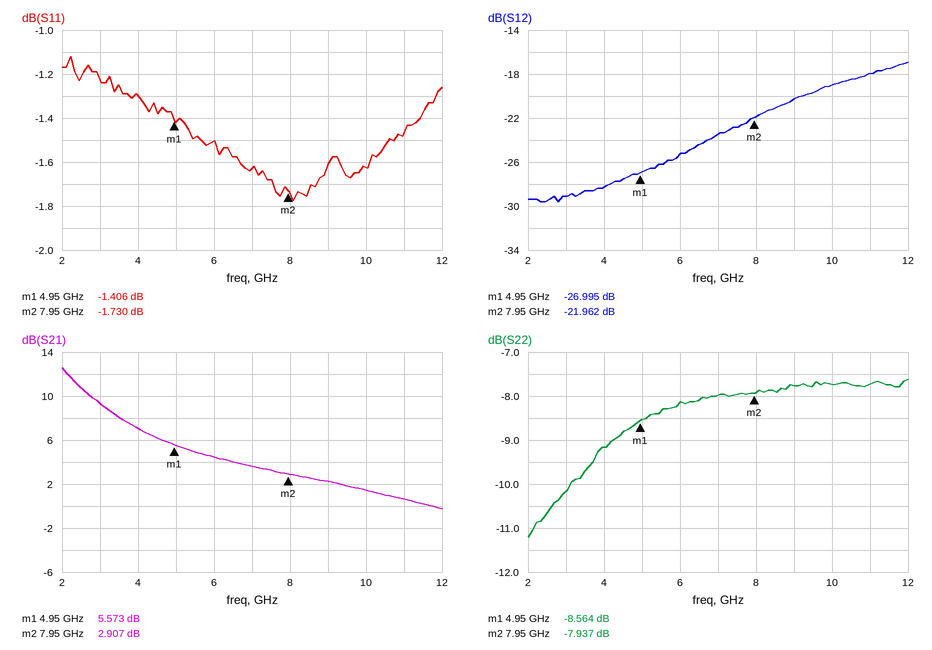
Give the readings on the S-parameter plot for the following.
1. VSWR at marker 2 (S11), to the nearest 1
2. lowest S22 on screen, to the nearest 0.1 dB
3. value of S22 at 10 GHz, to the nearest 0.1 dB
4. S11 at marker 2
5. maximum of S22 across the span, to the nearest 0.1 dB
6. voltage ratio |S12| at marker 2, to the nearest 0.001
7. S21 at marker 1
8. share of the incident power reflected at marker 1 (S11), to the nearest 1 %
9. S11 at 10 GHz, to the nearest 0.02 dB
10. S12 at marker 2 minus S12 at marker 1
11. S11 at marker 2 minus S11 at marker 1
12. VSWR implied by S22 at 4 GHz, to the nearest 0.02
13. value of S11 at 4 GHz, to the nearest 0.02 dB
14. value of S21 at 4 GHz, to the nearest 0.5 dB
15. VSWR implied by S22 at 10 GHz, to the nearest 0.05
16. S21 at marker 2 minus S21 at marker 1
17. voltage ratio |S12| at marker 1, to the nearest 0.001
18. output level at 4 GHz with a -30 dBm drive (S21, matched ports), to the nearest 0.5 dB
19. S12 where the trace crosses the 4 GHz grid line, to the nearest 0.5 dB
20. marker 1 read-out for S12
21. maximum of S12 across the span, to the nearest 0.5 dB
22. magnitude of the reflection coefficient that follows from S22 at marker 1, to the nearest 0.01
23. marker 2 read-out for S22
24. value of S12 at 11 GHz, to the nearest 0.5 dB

10
-11.2 dB
-7.7 dB
-1.730 dB
-7.6 dB
0.080
5.573 dB
72 %
-1.62 dB
5.033 dB
-0.324 dB
2.06
-1.30 dB
7.0 dB
2.40
-2.666 dB
0.045
-23.0 dBm
-28.5 dB
-26.995 dB
-17.0 dB
0.37
-7.937 dB
-18.0 dB
